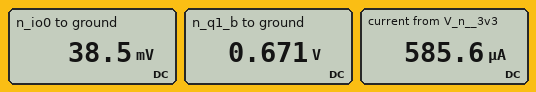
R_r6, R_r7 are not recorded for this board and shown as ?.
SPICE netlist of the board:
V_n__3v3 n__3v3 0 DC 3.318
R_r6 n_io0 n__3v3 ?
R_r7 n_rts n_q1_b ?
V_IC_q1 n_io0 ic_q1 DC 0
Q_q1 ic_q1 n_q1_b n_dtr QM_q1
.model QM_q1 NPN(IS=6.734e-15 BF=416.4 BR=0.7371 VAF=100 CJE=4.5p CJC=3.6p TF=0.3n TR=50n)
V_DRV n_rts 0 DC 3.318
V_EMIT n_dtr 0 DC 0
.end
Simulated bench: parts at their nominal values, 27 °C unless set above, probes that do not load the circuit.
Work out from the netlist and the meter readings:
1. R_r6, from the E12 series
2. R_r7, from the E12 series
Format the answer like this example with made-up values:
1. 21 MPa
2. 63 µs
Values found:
1. 5.6 kΩ
2. 6.8 kΩ
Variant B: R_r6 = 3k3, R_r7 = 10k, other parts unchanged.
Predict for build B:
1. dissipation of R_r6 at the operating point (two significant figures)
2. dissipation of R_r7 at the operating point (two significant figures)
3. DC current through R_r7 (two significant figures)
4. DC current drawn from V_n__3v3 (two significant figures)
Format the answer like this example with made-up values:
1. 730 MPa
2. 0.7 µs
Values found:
1. 3.2 mW
2. 700 µW
3. 260 µA
4. 990 µA
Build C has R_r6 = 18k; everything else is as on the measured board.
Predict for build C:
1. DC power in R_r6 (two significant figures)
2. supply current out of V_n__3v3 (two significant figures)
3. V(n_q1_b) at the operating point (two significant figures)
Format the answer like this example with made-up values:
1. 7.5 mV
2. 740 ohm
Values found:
1. 600 µW
2. 180 µA
3. 660 mV
